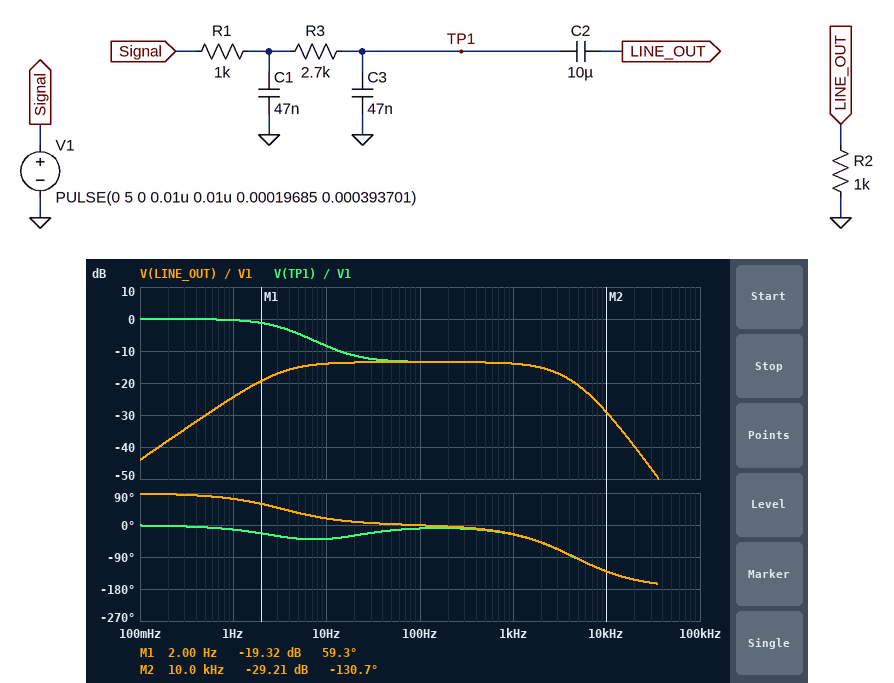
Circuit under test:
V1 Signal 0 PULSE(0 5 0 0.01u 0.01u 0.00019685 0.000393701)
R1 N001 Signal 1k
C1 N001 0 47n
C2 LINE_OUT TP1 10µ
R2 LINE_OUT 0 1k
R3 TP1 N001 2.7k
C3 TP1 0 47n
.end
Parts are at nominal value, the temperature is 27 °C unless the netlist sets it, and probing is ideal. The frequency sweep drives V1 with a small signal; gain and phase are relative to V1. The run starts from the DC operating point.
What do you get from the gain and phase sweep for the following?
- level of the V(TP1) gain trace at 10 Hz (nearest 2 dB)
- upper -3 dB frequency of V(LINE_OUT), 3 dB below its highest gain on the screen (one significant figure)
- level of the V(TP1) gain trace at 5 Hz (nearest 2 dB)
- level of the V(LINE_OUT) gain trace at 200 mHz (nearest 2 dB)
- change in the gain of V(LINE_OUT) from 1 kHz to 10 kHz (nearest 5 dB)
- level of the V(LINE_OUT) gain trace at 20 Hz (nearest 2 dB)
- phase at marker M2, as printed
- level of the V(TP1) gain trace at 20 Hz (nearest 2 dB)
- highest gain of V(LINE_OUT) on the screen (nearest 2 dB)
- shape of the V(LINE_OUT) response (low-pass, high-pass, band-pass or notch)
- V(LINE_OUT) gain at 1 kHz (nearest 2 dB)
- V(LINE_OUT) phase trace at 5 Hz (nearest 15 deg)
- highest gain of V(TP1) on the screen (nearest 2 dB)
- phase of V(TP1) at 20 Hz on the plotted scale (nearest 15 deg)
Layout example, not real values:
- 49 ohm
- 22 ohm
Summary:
- -8 dB
- 3 kHz
- -4 dB
- -38 dB
- -15 dB
- -14 dB
- -130.7 deg
- -12 dB
- -14 dB
- band-pass
- -14 dB
- 30 deg
- 0 dB
- -30 deg
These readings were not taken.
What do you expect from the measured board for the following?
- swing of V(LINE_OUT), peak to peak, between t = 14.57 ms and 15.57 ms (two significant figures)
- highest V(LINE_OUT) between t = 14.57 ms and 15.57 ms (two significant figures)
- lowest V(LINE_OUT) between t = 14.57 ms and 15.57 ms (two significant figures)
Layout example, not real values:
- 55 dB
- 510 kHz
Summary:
- 990 mV
- 880 mV
- -110 mV
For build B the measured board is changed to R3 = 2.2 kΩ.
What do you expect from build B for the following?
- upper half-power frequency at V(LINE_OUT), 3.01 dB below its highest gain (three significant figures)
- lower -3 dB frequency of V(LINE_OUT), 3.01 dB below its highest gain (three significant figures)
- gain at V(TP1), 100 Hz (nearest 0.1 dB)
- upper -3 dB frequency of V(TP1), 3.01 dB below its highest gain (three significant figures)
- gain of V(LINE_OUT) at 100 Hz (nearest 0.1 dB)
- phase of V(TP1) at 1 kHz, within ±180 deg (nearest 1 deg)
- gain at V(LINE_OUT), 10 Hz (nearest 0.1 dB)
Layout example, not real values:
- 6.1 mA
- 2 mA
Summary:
- 2.81 kHz
- 3.77 Hz
- -12.4 dB
- 4.01 Hz
- -12.5 dB
- -26 deg
- -13.1 dB
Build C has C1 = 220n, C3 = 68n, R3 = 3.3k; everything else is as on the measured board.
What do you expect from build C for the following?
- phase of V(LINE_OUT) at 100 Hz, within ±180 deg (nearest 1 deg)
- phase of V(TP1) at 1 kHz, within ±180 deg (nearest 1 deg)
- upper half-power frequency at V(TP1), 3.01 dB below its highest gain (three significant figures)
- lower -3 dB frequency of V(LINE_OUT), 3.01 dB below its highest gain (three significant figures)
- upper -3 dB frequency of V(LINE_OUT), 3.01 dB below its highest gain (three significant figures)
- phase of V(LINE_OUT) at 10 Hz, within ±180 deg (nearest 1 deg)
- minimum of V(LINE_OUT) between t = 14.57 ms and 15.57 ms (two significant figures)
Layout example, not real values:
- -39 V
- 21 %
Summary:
- -7 deg
- -67 deg
- 3.10 Hz
- 2.97 Hz
- 821 Hz
- 16 deg
- 190 mV
